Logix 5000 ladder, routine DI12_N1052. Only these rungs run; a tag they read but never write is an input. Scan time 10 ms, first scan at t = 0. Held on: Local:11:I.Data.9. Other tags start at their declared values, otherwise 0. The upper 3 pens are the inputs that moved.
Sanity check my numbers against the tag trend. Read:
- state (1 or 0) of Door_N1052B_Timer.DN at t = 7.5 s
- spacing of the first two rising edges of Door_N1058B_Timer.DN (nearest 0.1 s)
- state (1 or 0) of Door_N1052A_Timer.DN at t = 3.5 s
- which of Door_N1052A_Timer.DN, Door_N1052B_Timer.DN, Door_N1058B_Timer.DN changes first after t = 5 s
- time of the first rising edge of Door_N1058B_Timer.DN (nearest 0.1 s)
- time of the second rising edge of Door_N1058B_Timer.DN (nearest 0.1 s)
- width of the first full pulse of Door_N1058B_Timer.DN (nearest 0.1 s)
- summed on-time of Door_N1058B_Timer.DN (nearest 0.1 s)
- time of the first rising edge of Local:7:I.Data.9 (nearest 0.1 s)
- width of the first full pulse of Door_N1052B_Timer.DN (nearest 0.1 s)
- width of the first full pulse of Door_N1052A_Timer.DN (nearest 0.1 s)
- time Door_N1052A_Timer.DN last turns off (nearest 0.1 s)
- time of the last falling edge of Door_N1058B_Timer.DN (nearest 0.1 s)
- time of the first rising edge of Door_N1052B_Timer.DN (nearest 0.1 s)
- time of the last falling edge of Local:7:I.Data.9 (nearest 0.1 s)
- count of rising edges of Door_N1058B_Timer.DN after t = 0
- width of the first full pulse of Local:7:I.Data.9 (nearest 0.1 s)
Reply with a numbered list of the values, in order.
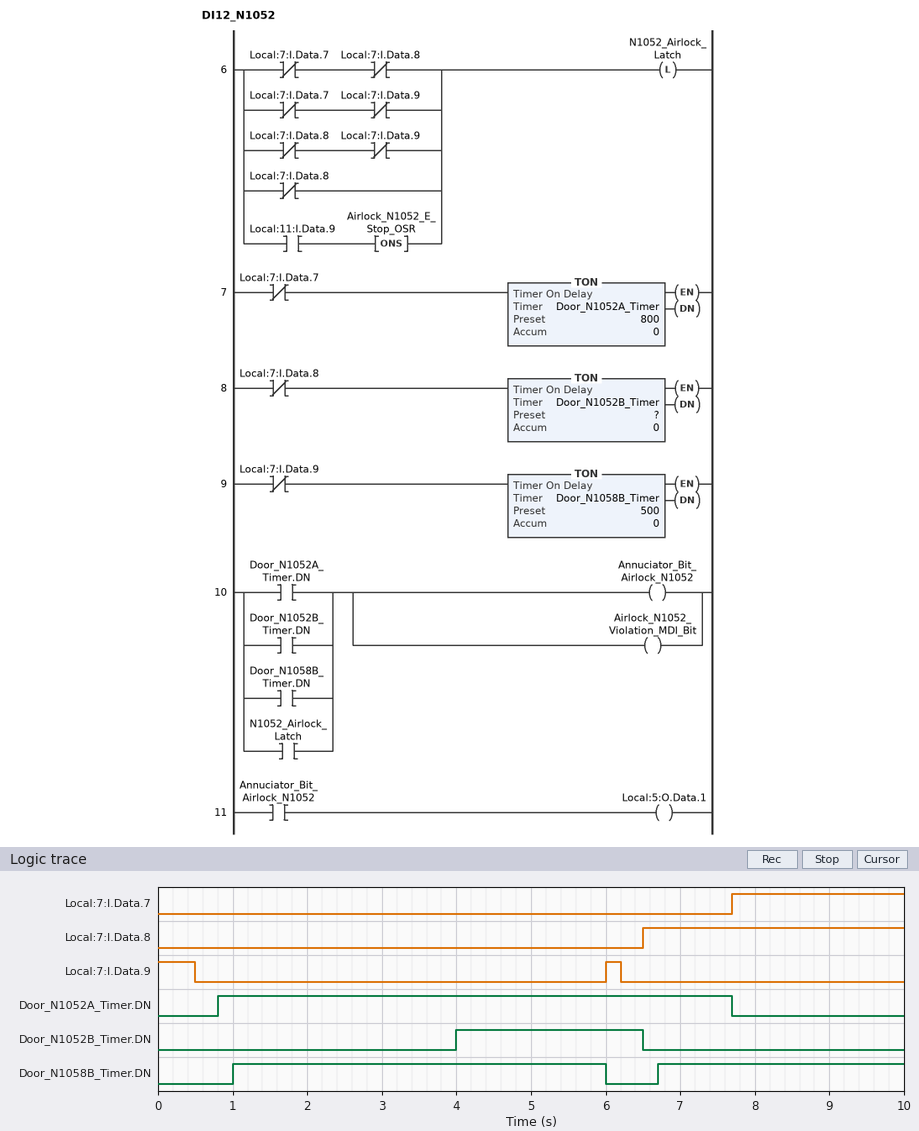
1. 0
2. 5.7 s
3. 1
4. Door_N1058B_Timer.DN
5. 1.0 s
6. 6.7 s
7. 5.0 s
8. 8.3 s
9. 6.0 s
10. 2.5 s
11. 6.9 s
12. 7.7 s
13. 6.0 s
14. 4.0 s
15. 6.2 s
16. 2
17. 0.2 s
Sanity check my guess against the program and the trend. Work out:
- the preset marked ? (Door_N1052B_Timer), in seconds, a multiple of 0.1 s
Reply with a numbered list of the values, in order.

1. 4.0 s
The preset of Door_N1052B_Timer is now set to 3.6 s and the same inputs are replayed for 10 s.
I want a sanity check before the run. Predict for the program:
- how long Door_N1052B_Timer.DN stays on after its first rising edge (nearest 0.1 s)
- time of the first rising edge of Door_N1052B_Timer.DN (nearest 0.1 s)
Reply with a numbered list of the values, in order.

1. 2.9 s
2. 3.6 s
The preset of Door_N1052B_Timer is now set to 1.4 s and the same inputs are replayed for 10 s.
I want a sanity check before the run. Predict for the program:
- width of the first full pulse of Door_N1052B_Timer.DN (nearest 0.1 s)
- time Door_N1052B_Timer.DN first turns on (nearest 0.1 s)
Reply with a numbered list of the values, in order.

1. 5.1 s
2. 1.4 s
